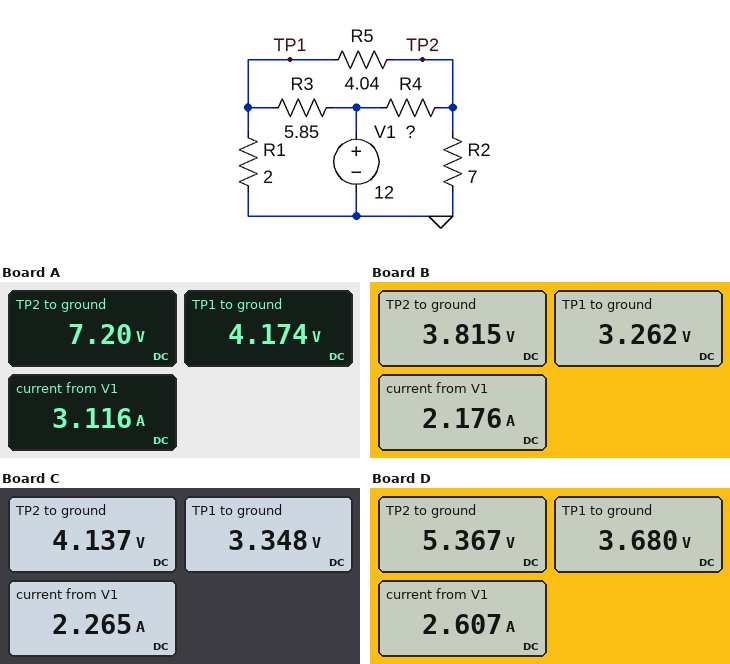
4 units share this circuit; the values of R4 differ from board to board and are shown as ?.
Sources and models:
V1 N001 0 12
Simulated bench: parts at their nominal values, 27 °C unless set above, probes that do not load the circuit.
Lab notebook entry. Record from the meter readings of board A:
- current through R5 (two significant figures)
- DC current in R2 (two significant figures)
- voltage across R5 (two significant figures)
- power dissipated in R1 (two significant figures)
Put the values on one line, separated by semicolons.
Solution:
750 mA; 1.0 A; 3.0 V; 8.7 W
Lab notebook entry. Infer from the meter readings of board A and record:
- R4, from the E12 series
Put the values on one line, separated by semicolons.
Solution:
2.7 Ω
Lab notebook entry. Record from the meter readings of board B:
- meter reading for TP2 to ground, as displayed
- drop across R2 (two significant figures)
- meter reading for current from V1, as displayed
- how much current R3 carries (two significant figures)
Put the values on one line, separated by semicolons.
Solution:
3.815 V; 3.8 V; 2.176 A; 1.5 A
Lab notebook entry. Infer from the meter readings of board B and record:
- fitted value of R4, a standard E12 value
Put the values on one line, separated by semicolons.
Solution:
12 Ω
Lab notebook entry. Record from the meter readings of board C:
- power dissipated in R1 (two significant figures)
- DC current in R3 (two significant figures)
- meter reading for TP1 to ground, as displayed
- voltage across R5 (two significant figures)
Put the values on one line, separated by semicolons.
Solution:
5.6 W; 1.5 A; 3.348 V; 790 mV
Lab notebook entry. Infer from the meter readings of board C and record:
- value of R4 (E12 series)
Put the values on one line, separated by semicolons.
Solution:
10 Ω
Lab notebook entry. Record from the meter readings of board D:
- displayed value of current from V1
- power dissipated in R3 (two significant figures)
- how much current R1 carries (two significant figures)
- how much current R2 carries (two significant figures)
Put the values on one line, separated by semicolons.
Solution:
2.607 A; 12 W; 1.8 A; 770 mA
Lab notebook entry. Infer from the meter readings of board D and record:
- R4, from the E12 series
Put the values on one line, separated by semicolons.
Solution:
5.6 Ω
